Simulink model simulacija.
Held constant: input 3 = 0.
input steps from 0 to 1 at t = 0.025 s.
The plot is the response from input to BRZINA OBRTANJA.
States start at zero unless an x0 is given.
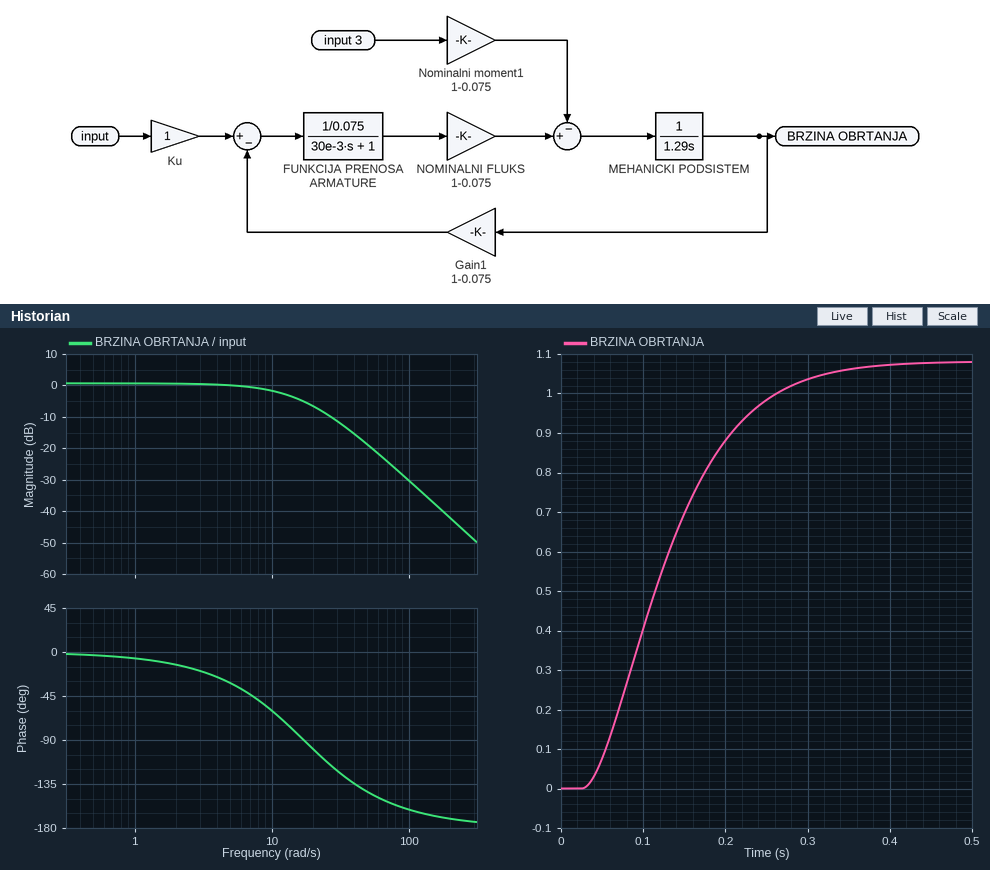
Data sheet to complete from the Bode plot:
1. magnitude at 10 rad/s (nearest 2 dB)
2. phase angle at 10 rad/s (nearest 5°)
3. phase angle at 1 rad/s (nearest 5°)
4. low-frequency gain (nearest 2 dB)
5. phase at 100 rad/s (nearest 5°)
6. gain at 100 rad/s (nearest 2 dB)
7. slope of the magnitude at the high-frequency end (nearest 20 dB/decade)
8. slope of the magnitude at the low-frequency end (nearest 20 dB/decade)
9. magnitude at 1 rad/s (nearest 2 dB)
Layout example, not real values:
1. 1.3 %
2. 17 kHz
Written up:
1. -2 dB
2. -60°
3. -5°
4. 0 dB
5. -160°
6. -30 dB
7. -40 dB/decade
8. 0 dB/decade
9. 0 dB
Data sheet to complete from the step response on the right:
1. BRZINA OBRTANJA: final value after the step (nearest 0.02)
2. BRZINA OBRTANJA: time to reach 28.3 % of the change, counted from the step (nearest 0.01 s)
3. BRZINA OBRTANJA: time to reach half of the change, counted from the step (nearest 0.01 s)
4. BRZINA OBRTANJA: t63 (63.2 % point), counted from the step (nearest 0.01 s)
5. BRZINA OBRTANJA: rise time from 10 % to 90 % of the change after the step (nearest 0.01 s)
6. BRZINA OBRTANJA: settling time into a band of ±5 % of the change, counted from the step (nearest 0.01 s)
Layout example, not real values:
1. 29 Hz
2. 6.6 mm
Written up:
1. 1.08
2. 0.06 s
3. 0.10 s
4. 0.12 s
5. 0.19 s
6. 0.26 s
